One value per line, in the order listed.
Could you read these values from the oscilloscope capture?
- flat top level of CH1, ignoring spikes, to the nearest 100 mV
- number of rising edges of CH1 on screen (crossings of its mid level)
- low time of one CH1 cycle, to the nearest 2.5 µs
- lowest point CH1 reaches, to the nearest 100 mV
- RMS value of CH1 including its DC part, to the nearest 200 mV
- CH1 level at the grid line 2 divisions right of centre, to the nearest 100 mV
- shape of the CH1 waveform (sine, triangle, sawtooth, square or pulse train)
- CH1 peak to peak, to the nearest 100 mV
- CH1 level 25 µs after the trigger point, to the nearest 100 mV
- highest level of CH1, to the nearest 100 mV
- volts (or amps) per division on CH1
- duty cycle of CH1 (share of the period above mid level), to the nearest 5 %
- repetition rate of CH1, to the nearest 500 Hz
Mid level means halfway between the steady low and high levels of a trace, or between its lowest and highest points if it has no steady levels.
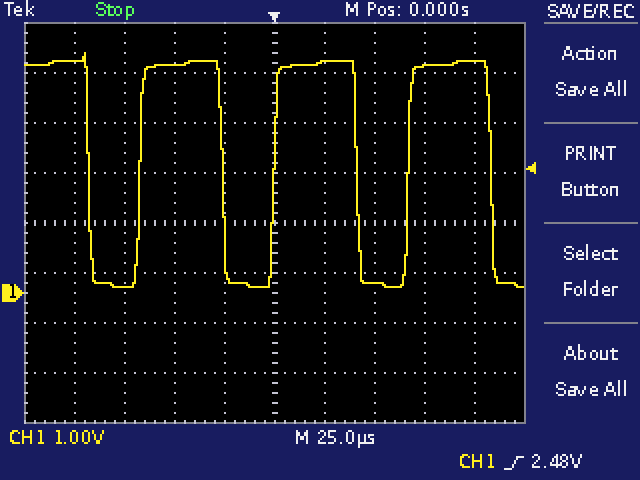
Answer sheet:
4.6 V
3
25.0 µs
100 mV
3.6 V
200 mV
pulse train
4.7 V
4.6 V
4.8 V
1 V
60 %
15.0 kHz
